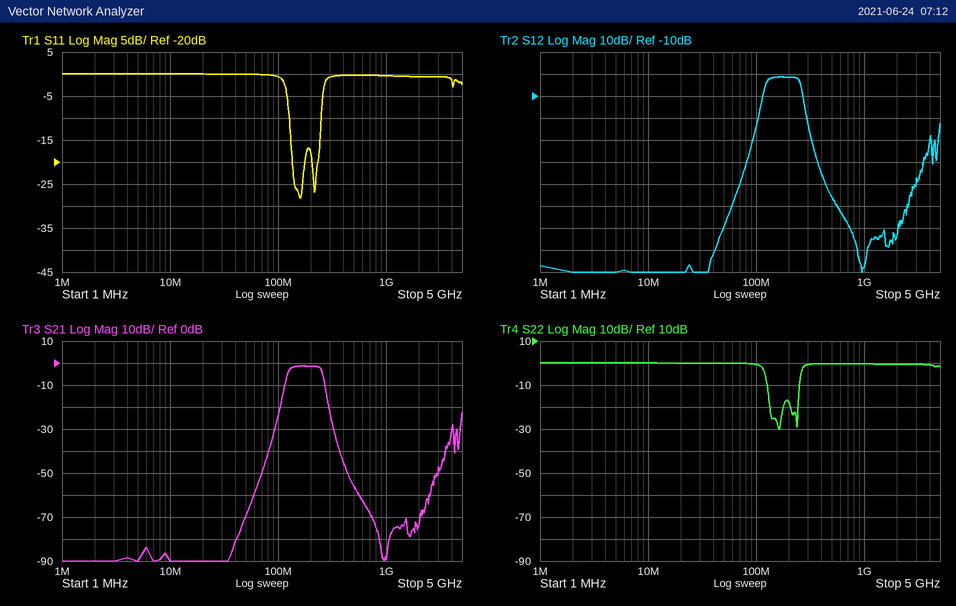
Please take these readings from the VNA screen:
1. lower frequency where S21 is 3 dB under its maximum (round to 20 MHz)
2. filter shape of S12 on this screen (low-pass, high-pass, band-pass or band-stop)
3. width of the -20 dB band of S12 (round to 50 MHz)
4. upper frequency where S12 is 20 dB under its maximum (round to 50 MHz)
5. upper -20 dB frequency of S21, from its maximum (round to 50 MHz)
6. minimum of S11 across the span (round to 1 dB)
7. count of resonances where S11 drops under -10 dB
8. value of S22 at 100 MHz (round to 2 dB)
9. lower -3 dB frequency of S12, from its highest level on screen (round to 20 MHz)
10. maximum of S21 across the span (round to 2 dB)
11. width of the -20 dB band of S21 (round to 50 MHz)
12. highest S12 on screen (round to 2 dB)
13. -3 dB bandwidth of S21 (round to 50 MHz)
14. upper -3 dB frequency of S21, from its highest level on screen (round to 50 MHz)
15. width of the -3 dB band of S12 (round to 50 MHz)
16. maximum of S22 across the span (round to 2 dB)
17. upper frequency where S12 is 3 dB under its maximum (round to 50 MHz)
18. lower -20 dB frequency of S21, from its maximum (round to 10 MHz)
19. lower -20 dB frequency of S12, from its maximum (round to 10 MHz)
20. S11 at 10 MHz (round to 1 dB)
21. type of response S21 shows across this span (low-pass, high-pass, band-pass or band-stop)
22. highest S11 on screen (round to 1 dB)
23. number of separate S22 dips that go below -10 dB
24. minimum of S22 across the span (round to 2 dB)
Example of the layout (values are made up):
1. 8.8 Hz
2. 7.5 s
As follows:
1. 120 MHz
2. band-pass
3. 200 MHz
4. 300 MHz
5. 300 MHz
6. -28 dB
7. 2
8. 0 dB
9. 120 MHz
10. -2 dB
11. 200 MHz
12. -2 dB
13. 150 MHz
14. 250 MHz
15. 150 MHz
16. 0 dB
17. 250 MHz
18. 100 MHz
19. 100 MHz
20. 0 dB
21. band-pass
22. 0 dB
23. 2
24. -30 dB
